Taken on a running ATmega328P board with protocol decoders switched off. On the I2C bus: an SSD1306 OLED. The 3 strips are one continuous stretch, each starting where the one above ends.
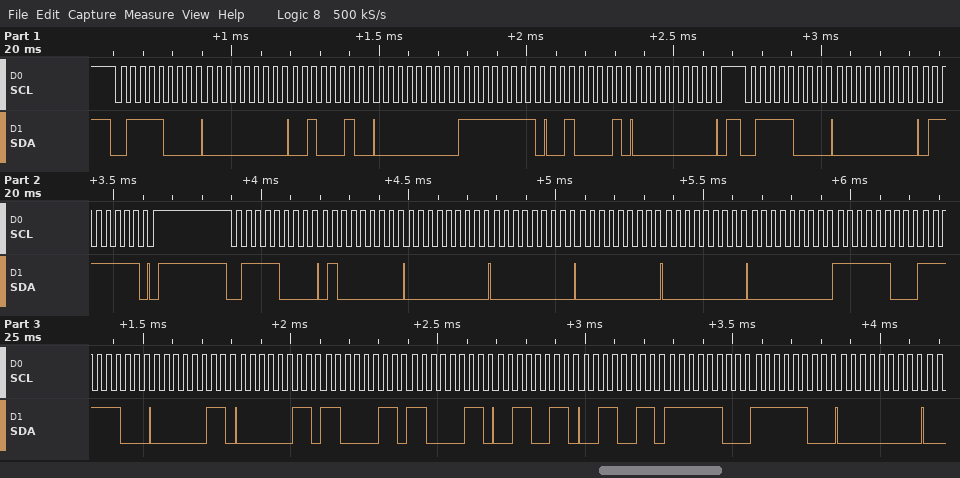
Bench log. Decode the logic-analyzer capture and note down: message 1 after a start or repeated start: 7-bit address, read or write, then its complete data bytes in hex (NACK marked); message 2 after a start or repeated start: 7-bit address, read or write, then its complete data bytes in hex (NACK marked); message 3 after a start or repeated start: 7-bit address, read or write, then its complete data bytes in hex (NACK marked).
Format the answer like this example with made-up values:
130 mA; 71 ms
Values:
0x3C write: 00 22 00 FF 21 00; 0x3C write: 00 7F; 0x3C write: 40 00 00 00 00 00 FC FC 03 03 C3 C3 33 33 FC FC 00
